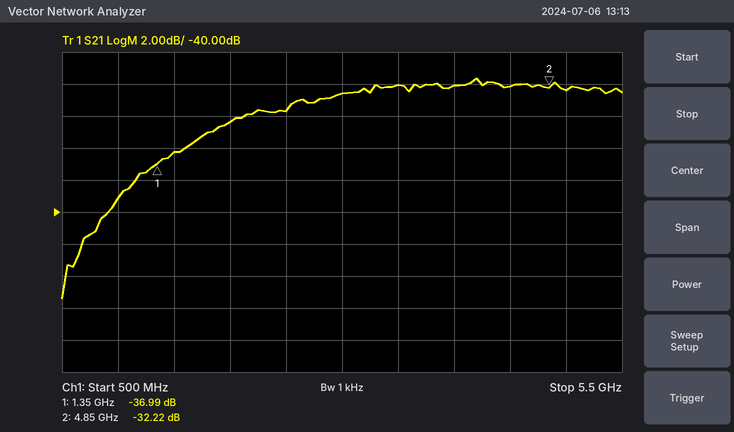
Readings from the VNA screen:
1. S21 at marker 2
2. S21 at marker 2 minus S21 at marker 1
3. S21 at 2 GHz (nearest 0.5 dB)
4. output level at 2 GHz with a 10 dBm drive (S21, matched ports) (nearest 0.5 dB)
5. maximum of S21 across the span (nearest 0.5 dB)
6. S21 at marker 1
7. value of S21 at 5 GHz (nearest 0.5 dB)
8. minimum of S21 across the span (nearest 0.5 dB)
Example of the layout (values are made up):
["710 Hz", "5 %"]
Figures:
["-32.22 dB", "4.77 dB", "-34.5 dB", "-24.5 dBm", "-31.5 dB", "-36.99 dB", "-32.5 dB", "-45.5 dB"]
